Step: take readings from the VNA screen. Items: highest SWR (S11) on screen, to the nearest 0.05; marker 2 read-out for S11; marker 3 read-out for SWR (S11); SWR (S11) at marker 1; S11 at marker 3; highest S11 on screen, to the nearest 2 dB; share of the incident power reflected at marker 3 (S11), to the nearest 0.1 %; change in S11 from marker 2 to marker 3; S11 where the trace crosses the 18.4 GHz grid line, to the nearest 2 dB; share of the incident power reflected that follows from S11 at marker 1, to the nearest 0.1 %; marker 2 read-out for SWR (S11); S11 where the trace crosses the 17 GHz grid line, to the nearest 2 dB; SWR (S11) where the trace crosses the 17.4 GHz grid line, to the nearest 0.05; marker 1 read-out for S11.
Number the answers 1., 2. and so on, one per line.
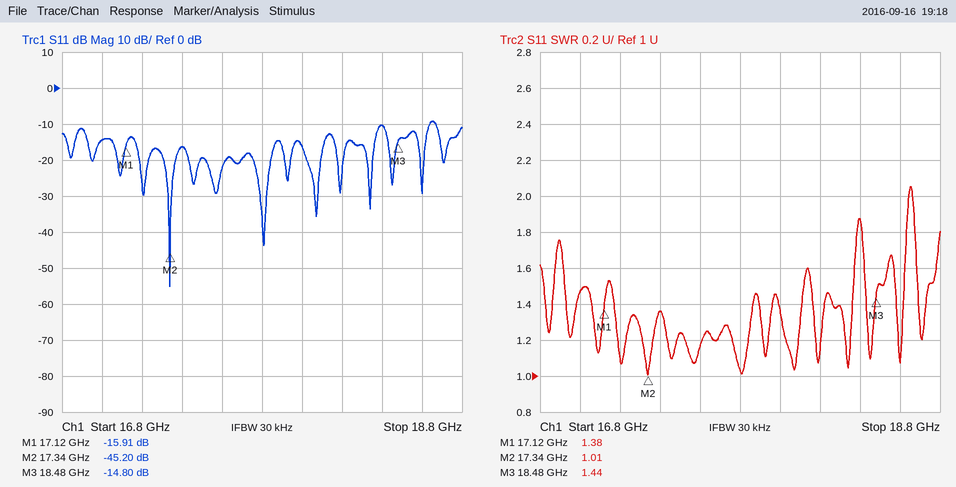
1. 2.05
2. -45.20 dB
3. 1.44
4. 1.38
5. -14.80 dB
6. -10 dB
7. 3.3 %
8. 30.40 dB
9. -10 dB
10. 2.6 %
11. 1.01
12. -14 dB
13. 1.35
14. -15.91 dB
